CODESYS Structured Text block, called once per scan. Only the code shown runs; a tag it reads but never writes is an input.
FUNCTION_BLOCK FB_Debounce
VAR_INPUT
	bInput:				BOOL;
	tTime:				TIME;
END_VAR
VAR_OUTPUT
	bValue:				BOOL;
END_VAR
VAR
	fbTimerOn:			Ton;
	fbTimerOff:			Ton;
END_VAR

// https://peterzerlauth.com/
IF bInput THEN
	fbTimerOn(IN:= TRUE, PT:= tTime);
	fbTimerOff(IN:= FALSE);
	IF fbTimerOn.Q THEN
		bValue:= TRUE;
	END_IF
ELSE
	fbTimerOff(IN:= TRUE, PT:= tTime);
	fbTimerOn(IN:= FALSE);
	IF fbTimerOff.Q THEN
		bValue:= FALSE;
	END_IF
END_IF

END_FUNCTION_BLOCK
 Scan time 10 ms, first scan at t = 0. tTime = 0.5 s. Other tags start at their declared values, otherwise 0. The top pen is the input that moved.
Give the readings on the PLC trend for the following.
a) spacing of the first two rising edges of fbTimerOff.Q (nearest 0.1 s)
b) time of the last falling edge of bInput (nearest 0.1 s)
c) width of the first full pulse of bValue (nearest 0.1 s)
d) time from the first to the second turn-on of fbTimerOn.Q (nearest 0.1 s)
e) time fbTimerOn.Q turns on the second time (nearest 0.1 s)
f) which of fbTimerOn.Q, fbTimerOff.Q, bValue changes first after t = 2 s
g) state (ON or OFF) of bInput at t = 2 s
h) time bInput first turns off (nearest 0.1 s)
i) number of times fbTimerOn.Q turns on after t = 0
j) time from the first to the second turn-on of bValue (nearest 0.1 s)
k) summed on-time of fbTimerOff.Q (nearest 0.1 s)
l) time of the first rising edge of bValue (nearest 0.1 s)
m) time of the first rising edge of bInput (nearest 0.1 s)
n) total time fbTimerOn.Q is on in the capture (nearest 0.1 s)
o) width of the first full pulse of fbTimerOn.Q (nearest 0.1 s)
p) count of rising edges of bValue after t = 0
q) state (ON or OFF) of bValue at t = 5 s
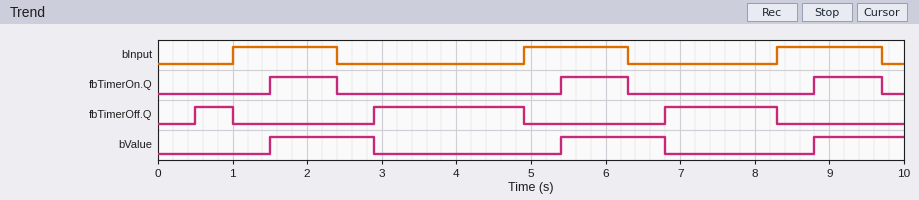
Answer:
2.4 s
9.7 s
1.4 s
3.9 s
5.4 s
fbTimerOn.Q
ON
2.4 s
3
3.9 s
4.0 s
1.5 s
1.0 s
2.7 s
0.9 s
3
OFF
